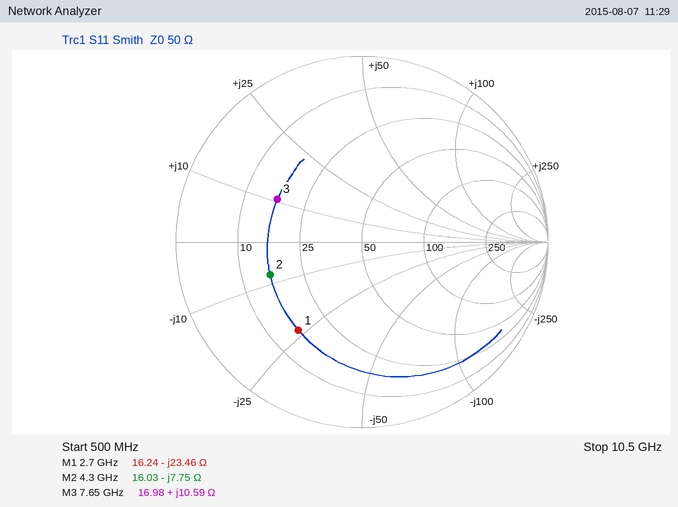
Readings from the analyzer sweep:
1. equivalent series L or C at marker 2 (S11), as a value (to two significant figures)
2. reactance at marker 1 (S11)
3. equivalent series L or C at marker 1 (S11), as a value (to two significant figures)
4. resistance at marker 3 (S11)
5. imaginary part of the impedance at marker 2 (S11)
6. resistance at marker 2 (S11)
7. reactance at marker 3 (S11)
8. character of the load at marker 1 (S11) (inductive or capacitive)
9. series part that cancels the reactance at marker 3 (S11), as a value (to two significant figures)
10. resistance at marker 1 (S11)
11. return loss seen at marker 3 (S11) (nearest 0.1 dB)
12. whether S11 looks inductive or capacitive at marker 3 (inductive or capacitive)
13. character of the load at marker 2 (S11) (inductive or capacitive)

4.8 pF
-23.46 Ω
2.5 pF
16.98 Ω
-7.75 Ω
16.03 Ω
+10.59 Ω
capacitive
2.0 pF
16.24 Ω
5.8 dB
inductive
capacitive
